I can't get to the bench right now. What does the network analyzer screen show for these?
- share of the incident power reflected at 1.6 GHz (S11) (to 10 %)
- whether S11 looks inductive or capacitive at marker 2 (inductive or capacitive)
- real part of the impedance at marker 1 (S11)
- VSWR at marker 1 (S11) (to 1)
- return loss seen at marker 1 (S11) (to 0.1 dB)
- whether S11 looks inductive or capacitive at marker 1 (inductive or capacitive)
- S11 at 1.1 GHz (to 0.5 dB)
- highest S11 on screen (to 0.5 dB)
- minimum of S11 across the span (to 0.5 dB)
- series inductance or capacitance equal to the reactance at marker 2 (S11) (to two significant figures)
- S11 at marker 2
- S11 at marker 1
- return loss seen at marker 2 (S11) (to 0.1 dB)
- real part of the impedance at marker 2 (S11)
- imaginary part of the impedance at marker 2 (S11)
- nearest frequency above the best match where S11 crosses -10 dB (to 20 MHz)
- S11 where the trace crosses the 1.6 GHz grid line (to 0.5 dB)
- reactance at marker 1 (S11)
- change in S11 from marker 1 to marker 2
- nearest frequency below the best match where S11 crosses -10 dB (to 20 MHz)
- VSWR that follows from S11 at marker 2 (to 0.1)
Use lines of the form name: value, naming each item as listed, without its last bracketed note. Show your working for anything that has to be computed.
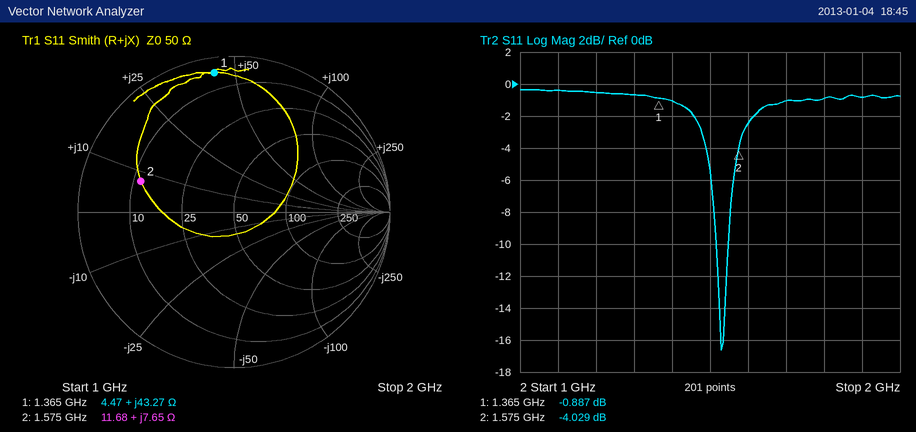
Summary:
share of the incident power reflected at 1.6 GHz (S11): 10^(-2.5/10) ≈ 56.2 %, so 60 % to the nearest 10 %
whether S11 looks inductive or capacitive at marker 2: inductive
real part of the impedance at marker 1: 4.47 Ω
VSWR at marker 1 (S11): (1 + 0.9029)/(1 − 0.9029) ≈ 20
return loss seen at marker 1 (S11): 0.9 dB
whether S11 looks inductive or capacitive at marker 1: inductive
S11 at 1.1 GHz: -0.5 dB
highest S11 on screen: -0.5 dB
minimum of S11 across the span: -16.5 dB
series inductance or capacitance equal to the reactance at marker 2 (S11): L = 7.65 Ω/(2π × 1.575 GHz) ≈ 773 pH, so 770 pH to two significant figures
S11 at marker 2: -4.029 dB
S11 at marker 1: -0.887 dB
return loss seen at marker 2 (S11): 4.0 dB
real part of the impedance at marker 2: 11.68 Ω
imaginary part of the impedance at marker 2: +7.65 Ω
nearest frequency above the best match where S11 crosses -10 dB: 1.54 GHz
S11 where the trace crosses the 1.6 GHz grid line: -2.5 dB
reactance at marker 1: +43.27 Ω
change in S11 from marker 1 to marker 2: -4.029 − (-0.887) = -3.142 dB
nearest frequency below the best match where S11 crosses -10 dB: 1.52 GHz
VSWR that follows from S11 at marker 2: (1 + 0.6289)/(1 − 0.6289) ≈ 4.4
